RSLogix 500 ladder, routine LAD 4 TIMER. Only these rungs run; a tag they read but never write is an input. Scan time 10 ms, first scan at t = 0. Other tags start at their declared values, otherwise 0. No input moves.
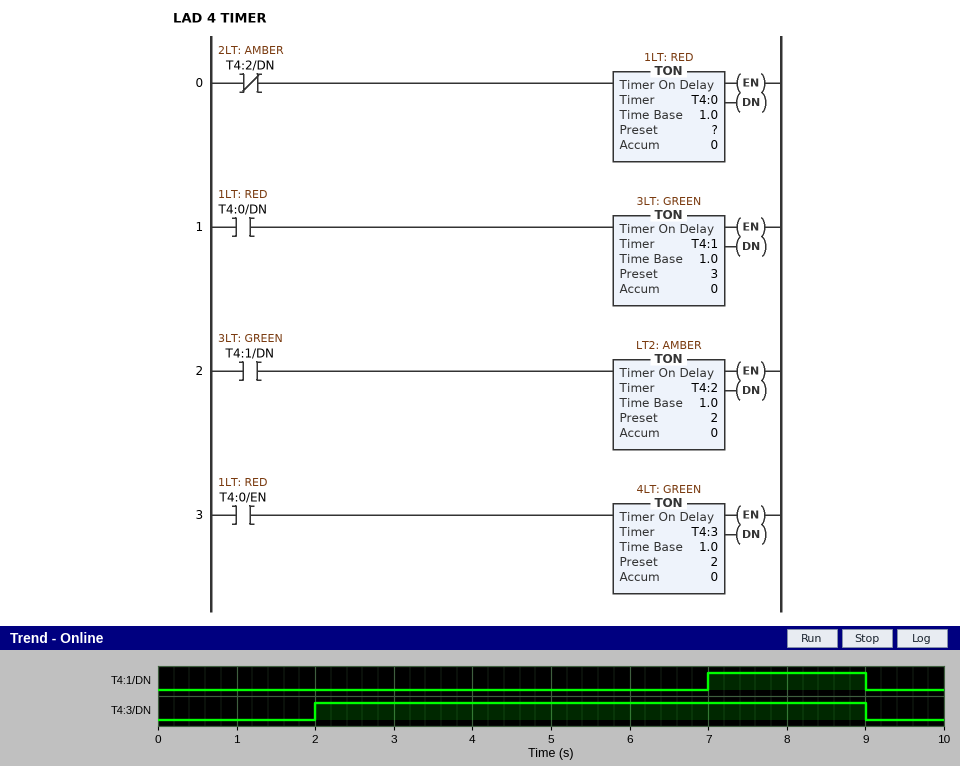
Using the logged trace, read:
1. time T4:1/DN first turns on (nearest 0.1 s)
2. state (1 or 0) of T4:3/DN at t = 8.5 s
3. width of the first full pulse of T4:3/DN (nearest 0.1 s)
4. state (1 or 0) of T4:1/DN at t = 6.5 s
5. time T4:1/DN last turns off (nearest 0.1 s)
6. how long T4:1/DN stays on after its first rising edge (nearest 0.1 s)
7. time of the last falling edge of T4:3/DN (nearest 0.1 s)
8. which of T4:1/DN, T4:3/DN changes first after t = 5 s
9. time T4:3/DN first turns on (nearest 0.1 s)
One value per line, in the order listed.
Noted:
7.0 s
1
7.0 s
0
9.0 s
2.0 s
9.0 s
T4:1/DN
2.0 s
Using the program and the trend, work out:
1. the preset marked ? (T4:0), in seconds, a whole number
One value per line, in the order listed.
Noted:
4 s
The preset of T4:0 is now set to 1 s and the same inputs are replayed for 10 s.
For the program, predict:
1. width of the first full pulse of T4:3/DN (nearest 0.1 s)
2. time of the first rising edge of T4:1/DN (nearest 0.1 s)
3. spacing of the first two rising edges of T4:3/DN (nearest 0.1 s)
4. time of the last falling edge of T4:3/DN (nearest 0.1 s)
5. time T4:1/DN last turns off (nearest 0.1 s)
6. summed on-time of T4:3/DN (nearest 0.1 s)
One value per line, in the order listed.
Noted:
4.0 s
4.0 s
6.0 s
6.0 s
6.0 s
6.0 s
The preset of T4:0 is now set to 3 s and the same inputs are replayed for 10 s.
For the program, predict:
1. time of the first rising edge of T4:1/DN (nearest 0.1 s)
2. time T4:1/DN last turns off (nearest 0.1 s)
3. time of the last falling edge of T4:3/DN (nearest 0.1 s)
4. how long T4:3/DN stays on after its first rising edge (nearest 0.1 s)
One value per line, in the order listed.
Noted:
6.0 s
8.0 s
8.0 s
6.0 s
